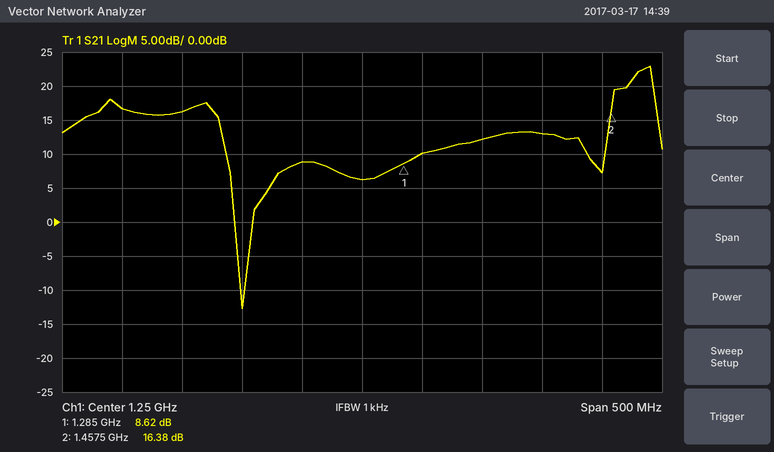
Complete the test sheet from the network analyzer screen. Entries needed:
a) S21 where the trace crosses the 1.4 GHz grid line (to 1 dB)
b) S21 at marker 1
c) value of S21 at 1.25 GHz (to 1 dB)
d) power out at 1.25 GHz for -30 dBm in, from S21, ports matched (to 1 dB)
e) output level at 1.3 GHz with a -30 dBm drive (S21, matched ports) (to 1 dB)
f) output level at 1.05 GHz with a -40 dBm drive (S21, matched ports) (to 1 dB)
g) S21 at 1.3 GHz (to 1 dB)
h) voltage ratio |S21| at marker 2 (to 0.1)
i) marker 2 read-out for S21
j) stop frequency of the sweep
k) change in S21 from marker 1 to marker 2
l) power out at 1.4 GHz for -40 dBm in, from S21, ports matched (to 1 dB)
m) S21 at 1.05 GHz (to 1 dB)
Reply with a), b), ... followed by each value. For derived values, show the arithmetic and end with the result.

a) 13 dB
b) 8.62 dB
c) 6 dB
d) -30 dBm + (6 dB) = -24 dBm
e) -30 dBm + (10 dB) = -20 dBm
f) -40 dBm + (17 dB) = -23 dBm
g) 10 dB
h) 10^(16.38/20) ≈ 6.6
i) 16.38 dB
j) 1.5 GHz
k) 16.38 − (8.62) = 7.76 dB
l) -40 dBm + (13 dB) = -27 dBm
m) 17 dB
